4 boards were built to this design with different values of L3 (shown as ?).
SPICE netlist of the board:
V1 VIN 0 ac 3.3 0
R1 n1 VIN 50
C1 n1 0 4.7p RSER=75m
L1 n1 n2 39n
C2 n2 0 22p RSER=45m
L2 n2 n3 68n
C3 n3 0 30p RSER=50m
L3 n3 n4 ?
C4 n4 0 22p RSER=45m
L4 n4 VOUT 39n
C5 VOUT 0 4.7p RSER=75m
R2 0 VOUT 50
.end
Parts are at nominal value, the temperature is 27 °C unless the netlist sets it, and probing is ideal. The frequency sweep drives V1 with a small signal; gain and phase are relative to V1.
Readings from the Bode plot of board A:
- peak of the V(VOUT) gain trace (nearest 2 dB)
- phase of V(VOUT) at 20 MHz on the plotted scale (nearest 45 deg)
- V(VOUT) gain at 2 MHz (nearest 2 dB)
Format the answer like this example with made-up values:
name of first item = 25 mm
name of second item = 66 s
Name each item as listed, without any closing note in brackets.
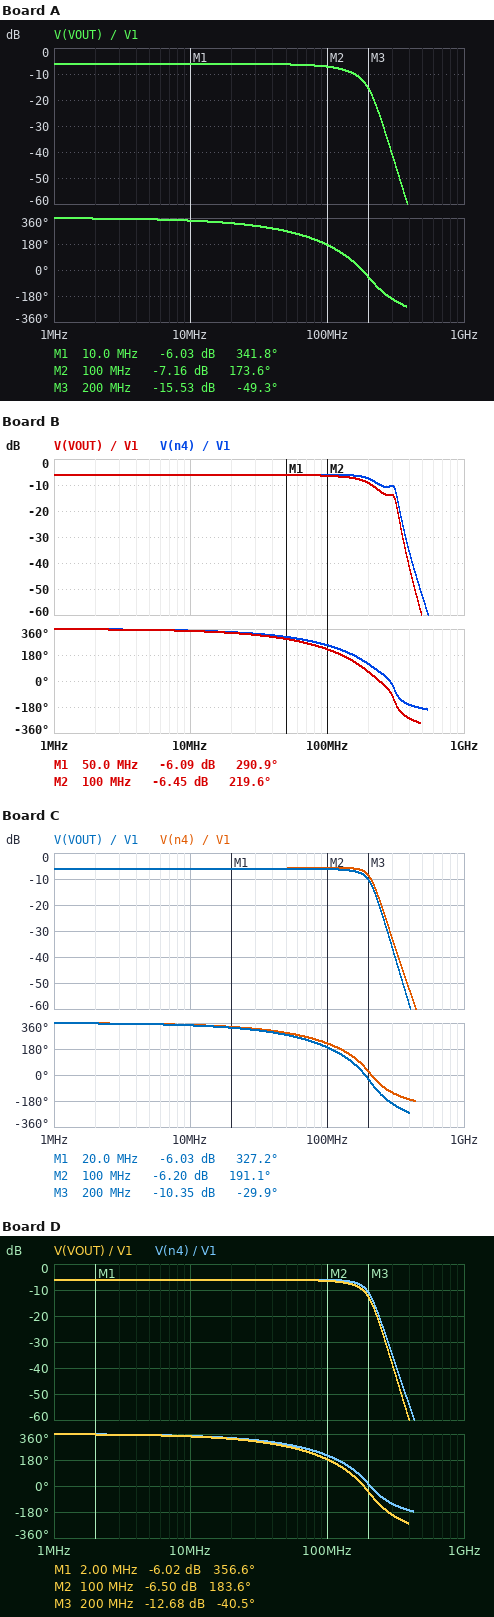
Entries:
peak of the V(VOUT) gain trace = -6 dB
phase of V(VOUT) at 20 MHz on the plotted scale = 315 deg
V(VOUT) gain at 2 MHz = -6 dB
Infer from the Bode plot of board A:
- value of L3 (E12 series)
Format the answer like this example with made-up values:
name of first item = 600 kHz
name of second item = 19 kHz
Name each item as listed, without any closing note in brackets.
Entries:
value of L3 = 150 nH
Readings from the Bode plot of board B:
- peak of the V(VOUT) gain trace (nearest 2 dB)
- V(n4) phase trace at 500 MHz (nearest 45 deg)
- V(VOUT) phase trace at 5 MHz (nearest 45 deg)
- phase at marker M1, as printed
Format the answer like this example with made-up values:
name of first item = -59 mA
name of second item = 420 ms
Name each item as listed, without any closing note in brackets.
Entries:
peak of the V(VOUT) gain trace = -6 dB
V(n4) phase trace at 500 MHz = -180 deg
V(VOUT) phase trace at 5 MHz = 360 deg
phase at marker M1, as printed = 290.9 deg
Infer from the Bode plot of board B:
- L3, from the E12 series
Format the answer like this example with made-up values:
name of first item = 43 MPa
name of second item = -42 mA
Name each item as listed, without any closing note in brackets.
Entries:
L3, from the E12 series = 27 nH
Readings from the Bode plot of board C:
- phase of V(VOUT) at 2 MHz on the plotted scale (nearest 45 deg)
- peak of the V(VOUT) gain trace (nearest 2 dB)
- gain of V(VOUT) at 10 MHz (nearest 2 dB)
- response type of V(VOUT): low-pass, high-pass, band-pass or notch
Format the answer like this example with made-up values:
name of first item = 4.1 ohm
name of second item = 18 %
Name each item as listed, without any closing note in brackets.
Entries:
phase of V(VOUT) at 2 MHz on the plotted scale = 360 deg
peak of the V(VOUT) gain trace = -6 dB
gain of V(VOUT) at 10 MHz = -6 dB
response type of V(VOUT): low-pass, high-pass, band-pass or notch = low-pass
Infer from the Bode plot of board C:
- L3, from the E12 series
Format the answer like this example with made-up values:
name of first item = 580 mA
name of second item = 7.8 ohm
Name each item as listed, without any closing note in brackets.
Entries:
L3, from the E12 series = 100 nH
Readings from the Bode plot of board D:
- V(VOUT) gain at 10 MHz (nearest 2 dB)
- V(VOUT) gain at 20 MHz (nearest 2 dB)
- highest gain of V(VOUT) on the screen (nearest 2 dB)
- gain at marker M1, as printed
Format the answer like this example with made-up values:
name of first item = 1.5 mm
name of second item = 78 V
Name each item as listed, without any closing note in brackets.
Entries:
V(VOUT) gain at 10 MHz = -6 dB
V(VOUT) gain at 20 MHz = -6 dB
highest gain of V(VOUT) on the screen = -6 dB
gain at marker M1, as printed = -6.02 dB
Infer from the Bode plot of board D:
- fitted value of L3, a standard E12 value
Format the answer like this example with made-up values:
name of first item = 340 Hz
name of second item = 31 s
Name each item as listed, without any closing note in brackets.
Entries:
fitted value of L3, a standard E12 value = 120 nH
